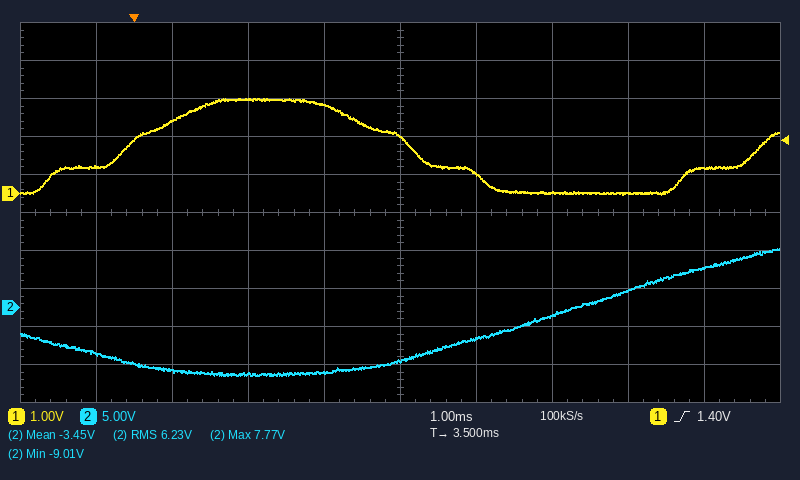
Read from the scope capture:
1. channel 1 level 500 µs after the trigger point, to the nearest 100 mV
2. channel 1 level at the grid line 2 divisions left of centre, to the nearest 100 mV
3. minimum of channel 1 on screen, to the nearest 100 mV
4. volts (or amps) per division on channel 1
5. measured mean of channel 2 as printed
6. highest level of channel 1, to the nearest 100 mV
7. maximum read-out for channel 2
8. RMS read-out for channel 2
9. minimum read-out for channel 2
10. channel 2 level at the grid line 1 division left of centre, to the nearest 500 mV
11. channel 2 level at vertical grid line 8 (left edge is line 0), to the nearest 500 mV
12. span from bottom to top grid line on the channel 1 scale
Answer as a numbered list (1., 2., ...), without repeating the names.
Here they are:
1. 1.9 V
2. 2.5 V
3. 0.0 V
4. 1 V
5. -3.45 V
6. 2.5 V
7. 7.77 V
8. 6.23 V
9. -9.01 V
10. -8.5 V
11. 2.5 V
12. 10 V
